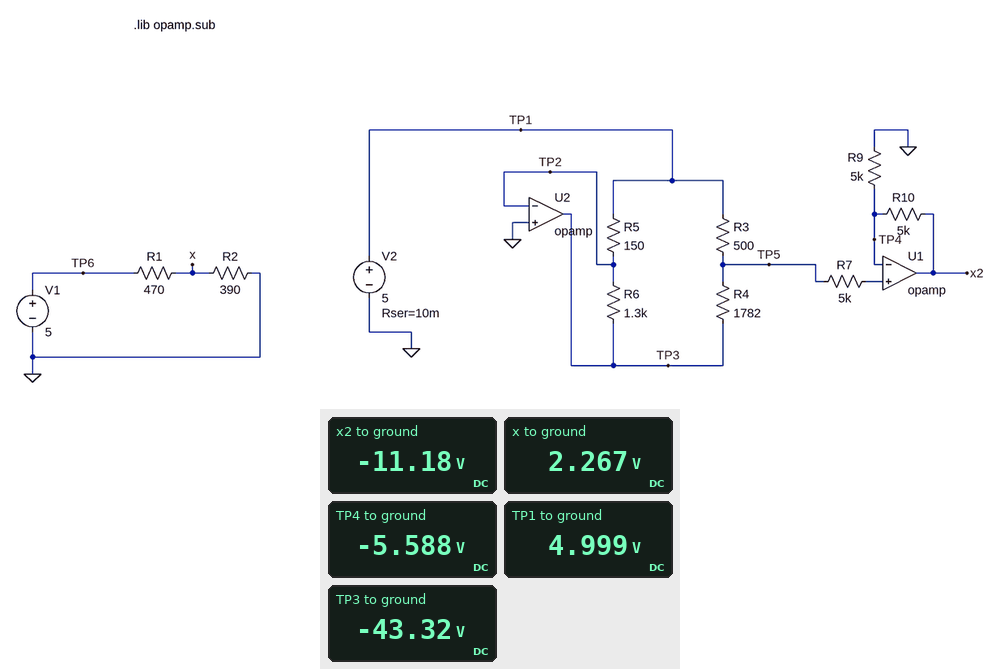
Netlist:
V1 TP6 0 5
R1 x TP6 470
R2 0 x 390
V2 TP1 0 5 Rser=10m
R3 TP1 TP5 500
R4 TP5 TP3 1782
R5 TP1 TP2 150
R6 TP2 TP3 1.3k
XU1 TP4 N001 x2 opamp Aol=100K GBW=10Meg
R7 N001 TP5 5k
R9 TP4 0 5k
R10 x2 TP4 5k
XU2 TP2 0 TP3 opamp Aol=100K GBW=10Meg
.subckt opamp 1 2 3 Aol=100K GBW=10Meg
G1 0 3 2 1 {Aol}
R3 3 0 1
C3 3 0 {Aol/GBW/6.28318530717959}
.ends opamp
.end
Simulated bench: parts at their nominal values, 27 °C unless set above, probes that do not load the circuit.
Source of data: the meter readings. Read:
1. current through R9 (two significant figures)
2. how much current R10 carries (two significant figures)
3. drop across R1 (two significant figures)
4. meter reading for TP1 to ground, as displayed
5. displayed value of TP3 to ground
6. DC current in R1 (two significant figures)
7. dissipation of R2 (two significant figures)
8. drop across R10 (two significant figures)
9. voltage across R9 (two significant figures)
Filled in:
1.1 mA
1.1 mA
2.7 V
4.999 V
-43.32 V
5.8 mA
13 mW
5.6 V
5.6 V
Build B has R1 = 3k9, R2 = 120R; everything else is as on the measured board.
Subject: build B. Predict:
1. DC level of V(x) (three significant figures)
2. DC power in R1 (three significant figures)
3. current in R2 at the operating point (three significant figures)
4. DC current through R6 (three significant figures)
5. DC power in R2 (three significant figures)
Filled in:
149 mV
6.03 mW
1.24 mA
33.3 mA
186 µW
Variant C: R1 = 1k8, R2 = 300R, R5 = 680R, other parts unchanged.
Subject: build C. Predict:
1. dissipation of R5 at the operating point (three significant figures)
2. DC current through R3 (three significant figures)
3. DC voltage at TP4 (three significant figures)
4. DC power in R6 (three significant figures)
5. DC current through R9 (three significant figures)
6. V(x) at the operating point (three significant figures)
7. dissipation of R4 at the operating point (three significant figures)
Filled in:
36.8 mW
6.38 mA
1.81 V
70.3 mW
362 µA
714 mV
72.5 mW
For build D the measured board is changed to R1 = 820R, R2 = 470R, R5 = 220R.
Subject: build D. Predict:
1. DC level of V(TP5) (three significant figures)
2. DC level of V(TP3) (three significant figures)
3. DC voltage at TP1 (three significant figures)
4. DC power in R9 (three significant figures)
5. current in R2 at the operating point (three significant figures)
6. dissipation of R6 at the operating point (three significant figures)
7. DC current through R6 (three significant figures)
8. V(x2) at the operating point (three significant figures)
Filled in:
-2.57 V
-29.5 V
5.00 V
1.32 mW
3.88 mA
671 mW
22.7 mA
-5.14 V
